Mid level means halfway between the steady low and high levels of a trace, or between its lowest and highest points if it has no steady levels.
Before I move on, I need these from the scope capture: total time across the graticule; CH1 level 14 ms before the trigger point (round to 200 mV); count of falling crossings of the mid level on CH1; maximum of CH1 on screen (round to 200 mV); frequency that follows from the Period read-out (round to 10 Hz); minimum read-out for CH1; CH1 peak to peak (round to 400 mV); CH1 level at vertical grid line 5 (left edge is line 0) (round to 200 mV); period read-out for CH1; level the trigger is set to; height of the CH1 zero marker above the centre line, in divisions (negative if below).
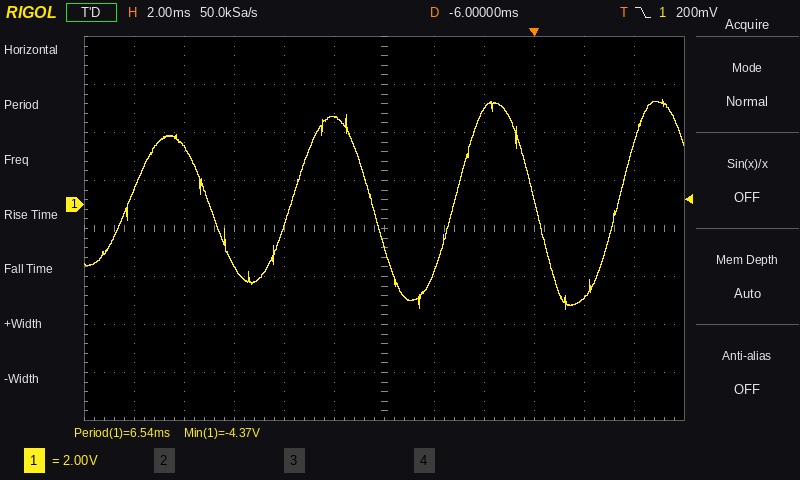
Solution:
24 ms
2.4 V
3
4.4 V
150 Hz
-4.37 V
8.8 V
3.6 V
6.54 ms
200 mV
+0.5 div
